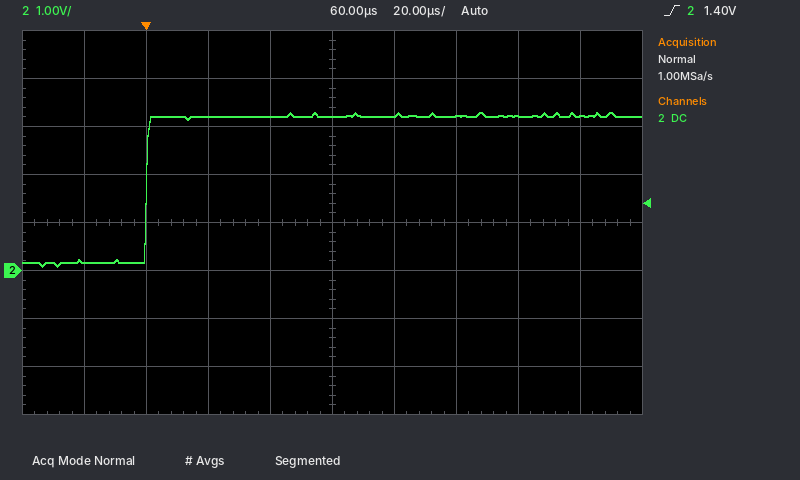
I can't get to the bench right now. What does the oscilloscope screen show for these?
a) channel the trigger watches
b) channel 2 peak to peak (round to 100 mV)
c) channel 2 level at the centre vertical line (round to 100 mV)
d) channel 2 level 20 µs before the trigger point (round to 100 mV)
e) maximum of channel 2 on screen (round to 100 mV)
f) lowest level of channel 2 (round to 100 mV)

channel 2
3.2 V
3.2 V
200 mV
3.3 V
100 mV
